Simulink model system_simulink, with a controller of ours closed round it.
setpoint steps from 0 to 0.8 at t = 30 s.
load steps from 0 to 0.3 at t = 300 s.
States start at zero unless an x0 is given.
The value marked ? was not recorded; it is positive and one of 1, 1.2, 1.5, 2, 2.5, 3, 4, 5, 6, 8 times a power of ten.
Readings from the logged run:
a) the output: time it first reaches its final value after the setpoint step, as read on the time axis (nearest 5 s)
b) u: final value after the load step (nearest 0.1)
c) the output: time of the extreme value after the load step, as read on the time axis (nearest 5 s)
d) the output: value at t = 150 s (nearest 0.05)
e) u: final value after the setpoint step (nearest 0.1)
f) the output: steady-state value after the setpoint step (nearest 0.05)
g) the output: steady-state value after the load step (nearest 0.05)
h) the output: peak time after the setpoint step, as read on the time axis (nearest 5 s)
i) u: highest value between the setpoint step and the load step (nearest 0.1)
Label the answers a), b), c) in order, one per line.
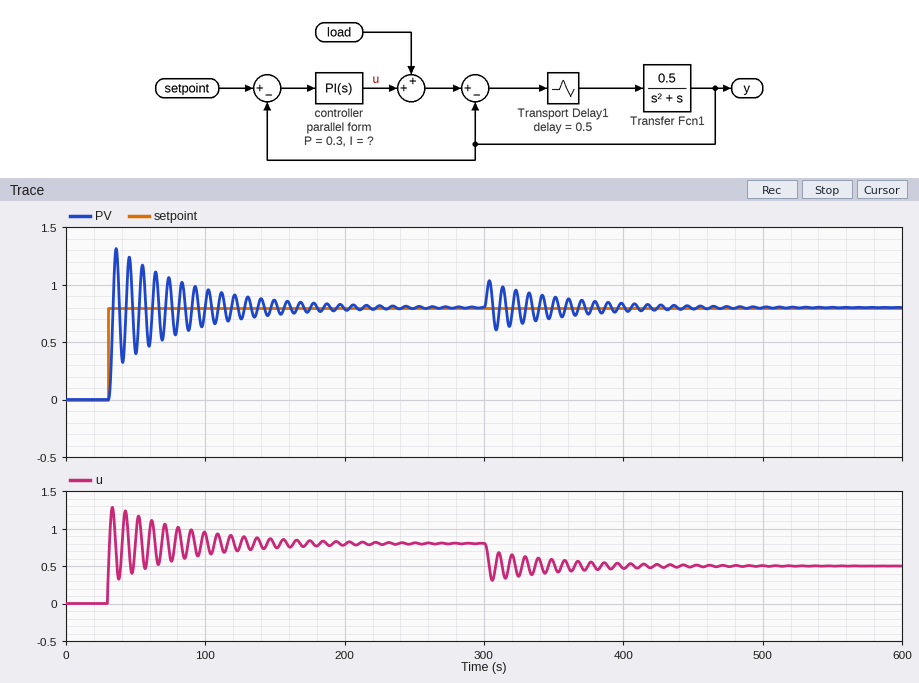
a) 35 s
b) 0.5
c) 305 s
d) 0.85
e) 0.8
f) 0.80
g) 0.80
h) 35 s
i) 1.3
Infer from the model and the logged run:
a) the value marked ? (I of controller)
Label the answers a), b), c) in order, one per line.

a) 0.6
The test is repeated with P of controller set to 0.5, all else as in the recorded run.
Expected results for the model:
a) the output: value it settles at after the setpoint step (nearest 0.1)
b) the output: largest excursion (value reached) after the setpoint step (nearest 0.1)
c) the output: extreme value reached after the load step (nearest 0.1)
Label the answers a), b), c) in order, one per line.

a) 0.8
b) 1.2
c) 1.0
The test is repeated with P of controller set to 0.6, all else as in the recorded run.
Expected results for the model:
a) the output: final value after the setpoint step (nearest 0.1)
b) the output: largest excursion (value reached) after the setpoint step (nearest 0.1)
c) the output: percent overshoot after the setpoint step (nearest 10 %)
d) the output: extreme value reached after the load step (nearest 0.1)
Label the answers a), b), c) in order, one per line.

a) 0.8
b) 1.2
c) 50 %
d) 1.0
